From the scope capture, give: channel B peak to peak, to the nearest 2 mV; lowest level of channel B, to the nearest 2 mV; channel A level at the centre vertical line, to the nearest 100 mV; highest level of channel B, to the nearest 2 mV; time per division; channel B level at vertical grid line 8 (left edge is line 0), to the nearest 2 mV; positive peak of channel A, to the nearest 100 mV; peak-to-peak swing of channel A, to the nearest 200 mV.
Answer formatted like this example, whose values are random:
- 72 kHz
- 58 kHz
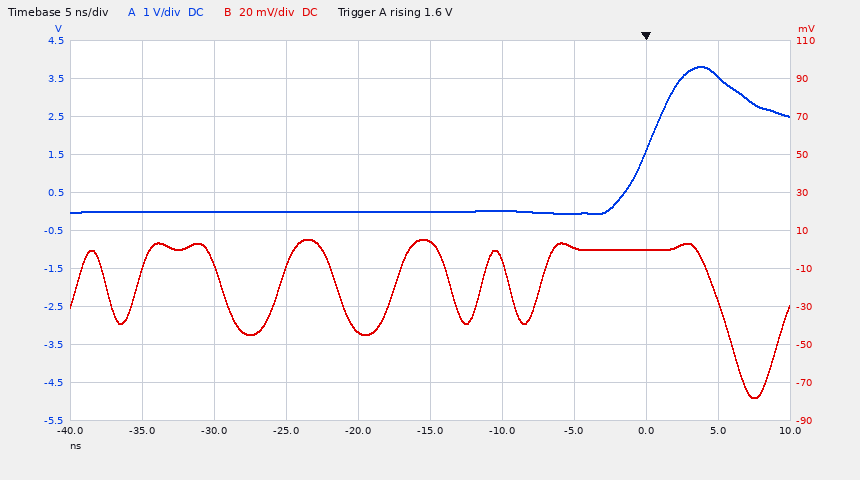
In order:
- 84 mV
- -78 mV
- 0.0 V
- 6 mV
- 5 ns
- 0 mV
- 3.8 V
- 3.8 V
